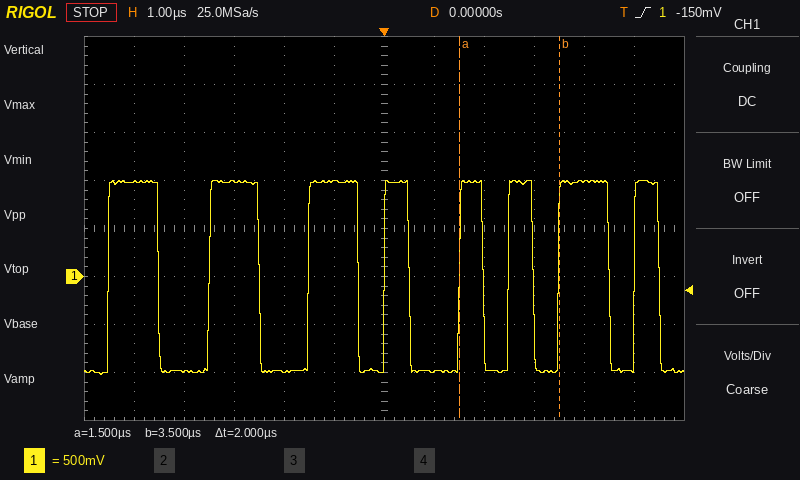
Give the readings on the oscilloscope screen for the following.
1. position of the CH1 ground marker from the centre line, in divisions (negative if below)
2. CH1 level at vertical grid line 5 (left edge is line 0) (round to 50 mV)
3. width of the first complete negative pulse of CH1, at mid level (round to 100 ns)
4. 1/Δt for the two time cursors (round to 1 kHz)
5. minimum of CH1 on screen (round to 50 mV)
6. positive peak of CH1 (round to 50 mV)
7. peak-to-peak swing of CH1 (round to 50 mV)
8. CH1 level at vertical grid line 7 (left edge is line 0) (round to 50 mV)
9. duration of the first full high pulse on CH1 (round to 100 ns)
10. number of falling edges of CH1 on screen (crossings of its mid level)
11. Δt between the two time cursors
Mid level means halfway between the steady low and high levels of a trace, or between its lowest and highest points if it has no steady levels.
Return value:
-1.0 div
1.00 V
1.0 µs
500 kHz
-1.00 V
1.00 V
2.00 V
-1.00 V
1.0 µs
8
2 µs
